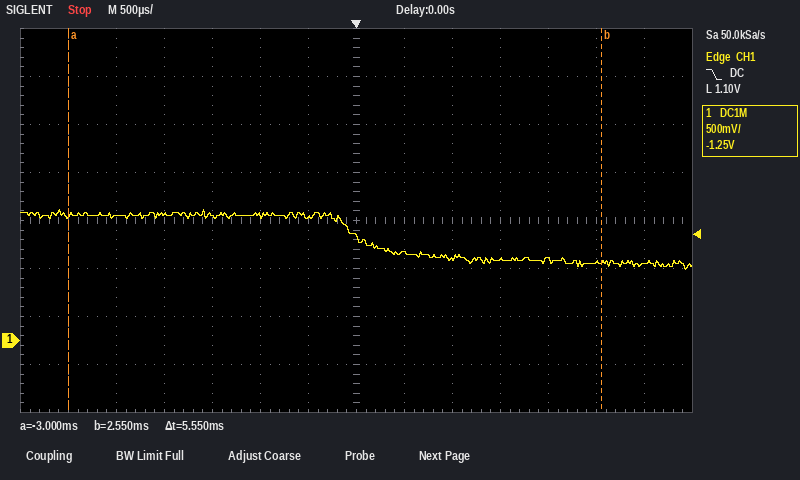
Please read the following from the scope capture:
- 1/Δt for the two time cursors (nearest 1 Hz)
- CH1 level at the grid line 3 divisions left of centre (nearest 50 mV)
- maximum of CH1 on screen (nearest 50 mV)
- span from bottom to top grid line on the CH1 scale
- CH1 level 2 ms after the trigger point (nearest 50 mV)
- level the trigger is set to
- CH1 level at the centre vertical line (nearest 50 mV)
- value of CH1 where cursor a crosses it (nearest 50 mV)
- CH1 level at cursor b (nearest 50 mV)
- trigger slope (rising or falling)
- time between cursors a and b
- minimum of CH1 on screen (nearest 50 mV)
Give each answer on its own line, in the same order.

180 Hz
1.30 V
1.35 V
4 V
850 mV
1.10 V
1.10 V
1.30 V
800 mV
falling
5.55 ms
750 mV
